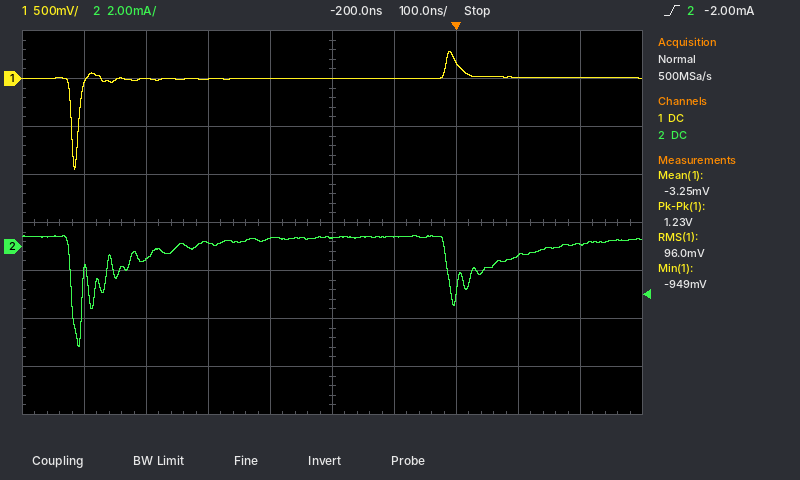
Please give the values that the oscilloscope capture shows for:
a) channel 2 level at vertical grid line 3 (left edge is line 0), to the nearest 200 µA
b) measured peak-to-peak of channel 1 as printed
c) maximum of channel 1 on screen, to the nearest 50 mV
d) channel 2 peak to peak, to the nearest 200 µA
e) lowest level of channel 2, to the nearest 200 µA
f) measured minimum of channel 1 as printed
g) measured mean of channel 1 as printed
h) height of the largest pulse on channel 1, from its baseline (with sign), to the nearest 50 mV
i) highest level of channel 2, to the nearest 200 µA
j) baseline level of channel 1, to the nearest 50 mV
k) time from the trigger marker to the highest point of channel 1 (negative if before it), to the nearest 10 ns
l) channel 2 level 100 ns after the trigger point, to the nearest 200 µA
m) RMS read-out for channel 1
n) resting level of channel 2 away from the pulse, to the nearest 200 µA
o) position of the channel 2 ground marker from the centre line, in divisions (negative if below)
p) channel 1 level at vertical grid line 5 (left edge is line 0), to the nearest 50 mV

200 µA
1.23 V
300 mV
4.6 mA
-4.2 mA
-949 mV
-3.25 mV
-950 mV
400 µA
0 mV
-10 ns
-400 µA
96.0 mV
400 µA
-0.5 div
0 mV
